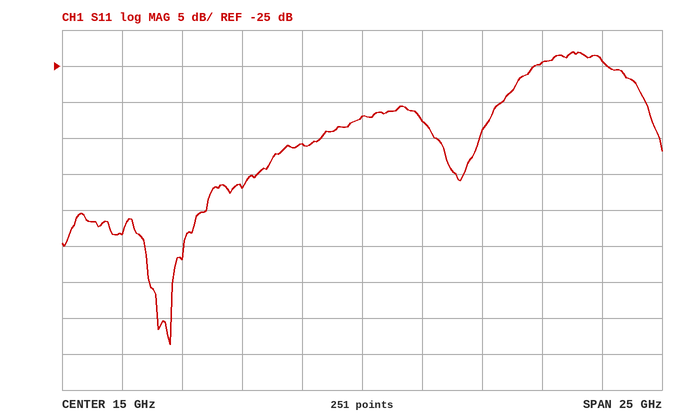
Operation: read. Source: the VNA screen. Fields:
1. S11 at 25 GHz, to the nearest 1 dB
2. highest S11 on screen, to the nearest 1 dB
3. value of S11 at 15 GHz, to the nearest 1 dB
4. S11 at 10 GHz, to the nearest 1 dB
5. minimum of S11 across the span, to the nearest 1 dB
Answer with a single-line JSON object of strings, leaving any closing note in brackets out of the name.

{"S11 at 25 GHz, to the nearest 1 dB": "-24 dB", "highest S11 on screen, to the nearest 1 dB": "-23 dB", "value of S11 at 15 GHz, to the nearest 1 dB": "-32 dB", "S11 at 10 GHz, to the nearest 1 dB": "-42 dB", "minimum of S11 across the span, to the nearest 1 dB": "-64 dB"}
